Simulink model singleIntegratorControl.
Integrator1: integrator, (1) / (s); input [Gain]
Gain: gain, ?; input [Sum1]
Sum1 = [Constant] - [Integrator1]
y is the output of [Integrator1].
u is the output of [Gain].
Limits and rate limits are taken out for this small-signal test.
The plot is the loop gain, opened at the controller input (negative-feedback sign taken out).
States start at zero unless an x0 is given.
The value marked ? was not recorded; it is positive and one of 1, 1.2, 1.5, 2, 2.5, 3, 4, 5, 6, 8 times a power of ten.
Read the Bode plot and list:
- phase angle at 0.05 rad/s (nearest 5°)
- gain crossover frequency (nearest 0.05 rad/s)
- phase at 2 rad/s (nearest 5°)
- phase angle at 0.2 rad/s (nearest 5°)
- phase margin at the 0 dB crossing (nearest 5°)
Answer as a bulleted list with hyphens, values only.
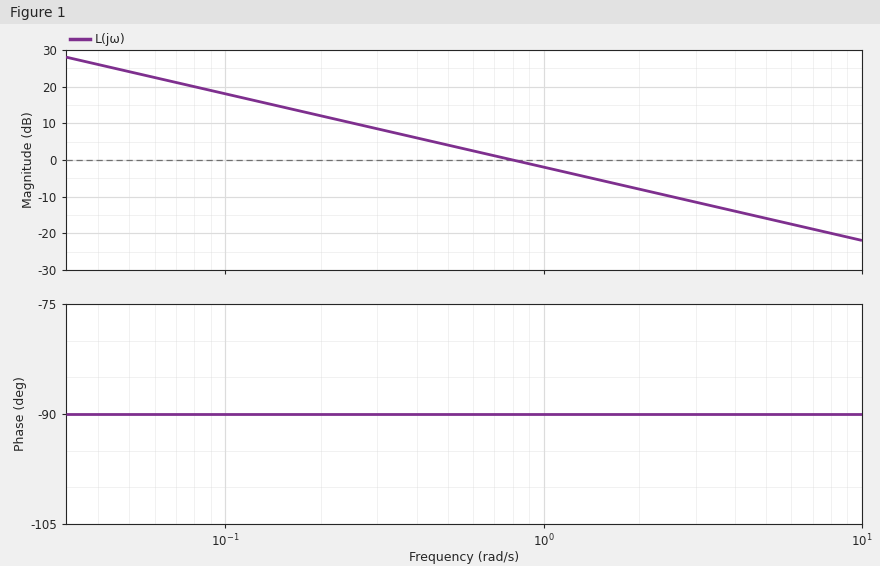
- -90°
- 0.80 rad/s
- -90°
- -90°
- 90°
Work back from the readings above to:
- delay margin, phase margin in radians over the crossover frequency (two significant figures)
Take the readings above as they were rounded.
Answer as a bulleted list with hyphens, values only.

- 2.0 s
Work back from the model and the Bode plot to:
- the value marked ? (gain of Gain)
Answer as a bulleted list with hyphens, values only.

- 0.8
